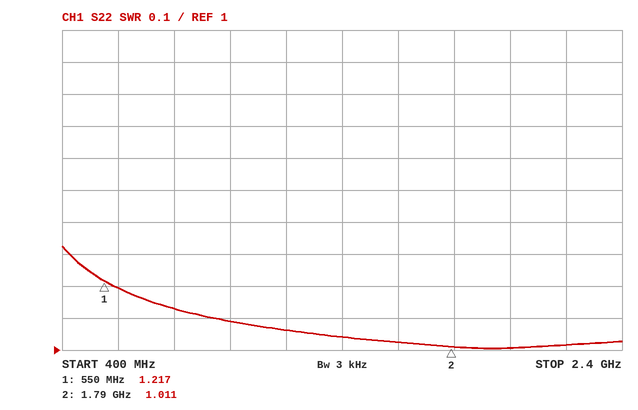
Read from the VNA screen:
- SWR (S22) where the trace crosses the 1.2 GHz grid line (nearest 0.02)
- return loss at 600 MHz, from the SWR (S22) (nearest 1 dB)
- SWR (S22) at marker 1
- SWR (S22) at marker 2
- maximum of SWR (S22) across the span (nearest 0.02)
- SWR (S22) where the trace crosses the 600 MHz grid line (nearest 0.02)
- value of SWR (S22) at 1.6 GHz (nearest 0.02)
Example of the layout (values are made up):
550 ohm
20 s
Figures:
1.06
21 dB
1.217
1.011
1.32
1.20
1.02
